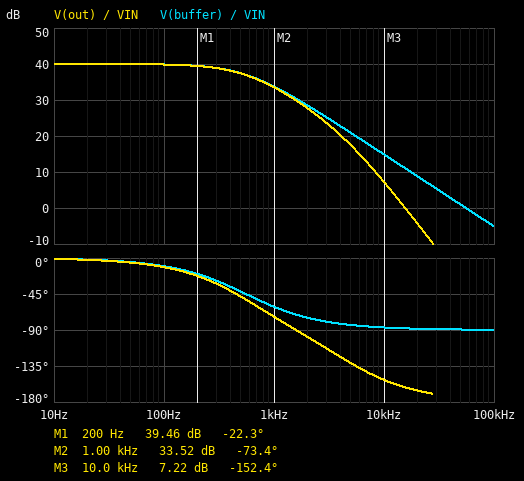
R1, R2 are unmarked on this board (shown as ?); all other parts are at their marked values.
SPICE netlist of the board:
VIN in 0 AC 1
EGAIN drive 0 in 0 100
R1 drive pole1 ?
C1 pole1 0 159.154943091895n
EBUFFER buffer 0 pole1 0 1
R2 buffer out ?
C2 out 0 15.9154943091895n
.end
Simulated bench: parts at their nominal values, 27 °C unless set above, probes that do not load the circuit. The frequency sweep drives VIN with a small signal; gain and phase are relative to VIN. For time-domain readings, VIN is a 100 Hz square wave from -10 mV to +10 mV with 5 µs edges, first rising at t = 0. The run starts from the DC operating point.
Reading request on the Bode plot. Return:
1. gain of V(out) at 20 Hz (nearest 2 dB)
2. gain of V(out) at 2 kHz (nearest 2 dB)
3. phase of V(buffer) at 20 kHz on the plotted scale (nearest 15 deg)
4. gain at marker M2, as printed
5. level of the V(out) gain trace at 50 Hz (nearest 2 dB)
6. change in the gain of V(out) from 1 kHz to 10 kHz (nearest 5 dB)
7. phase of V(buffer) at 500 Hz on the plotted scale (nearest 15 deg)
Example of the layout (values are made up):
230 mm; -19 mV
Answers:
40 dB; 28 dB; -90 deg; 33.52 dB; 40 dB; -25 dB; -45 deg
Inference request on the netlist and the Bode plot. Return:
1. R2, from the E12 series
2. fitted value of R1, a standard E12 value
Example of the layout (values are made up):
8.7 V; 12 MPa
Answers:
2.2 kΩ; 1.8 kΩ
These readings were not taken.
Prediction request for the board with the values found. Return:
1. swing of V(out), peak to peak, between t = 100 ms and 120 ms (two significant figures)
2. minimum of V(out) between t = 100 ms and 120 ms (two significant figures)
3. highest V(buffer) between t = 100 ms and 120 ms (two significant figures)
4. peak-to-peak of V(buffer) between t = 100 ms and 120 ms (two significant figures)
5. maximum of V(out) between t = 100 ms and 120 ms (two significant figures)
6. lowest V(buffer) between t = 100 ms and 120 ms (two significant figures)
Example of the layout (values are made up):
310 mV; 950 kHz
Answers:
2.0 V; -1.0 V; 1.0 V; 2.0 V; 1.0 V; -1.0 V
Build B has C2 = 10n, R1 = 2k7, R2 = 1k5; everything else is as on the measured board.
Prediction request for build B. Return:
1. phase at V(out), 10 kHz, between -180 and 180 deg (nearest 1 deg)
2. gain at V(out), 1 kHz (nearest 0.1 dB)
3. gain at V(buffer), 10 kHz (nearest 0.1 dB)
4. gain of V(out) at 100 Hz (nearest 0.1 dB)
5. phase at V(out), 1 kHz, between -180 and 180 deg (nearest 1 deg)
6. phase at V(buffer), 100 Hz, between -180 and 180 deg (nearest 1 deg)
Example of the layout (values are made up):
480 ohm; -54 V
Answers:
-131 deg; 30.8 dB; 11.4 dB; 39.7 dB; -75 deg; -15 deg
